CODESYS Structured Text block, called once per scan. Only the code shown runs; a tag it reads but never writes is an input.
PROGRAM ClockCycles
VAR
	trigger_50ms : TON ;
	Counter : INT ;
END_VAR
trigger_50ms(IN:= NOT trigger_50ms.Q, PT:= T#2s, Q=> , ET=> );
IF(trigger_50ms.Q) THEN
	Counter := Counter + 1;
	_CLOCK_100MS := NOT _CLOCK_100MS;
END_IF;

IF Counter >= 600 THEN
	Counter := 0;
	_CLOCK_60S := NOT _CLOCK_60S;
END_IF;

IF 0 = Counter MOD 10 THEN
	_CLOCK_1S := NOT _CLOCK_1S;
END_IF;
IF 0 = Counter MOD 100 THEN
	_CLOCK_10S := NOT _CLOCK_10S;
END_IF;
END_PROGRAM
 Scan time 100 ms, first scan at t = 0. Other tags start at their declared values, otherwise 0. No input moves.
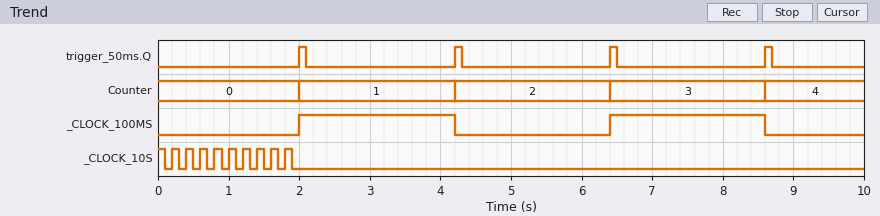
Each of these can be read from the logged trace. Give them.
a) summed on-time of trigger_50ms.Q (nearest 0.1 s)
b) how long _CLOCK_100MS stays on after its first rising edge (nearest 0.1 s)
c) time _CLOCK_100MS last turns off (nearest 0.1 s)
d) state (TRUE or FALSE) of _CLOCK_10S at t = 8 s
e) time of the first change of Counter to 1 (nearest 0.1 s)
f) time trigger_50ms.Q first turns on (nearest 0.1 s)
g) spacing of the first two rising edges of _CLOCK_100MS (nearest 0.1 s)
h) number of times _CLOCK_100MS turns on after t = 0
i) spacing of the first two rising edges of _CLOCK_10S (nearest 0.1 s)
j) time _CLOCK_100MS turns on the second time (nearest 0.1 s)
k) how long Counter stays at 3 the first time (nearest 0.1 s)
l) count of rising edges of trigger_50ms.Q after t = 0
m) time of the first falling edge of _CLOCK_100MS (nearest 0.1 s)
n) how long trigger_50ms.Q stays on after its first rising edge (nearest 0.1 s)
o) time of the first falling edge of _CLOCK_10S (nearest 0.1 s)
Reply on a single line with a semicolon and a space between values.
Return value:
0.4 s; 2.2 s; 8.6 s; FALSE; 2.0 s; 2.0 s; 4.4 s; 2; 0.2 s; 6.4 s; 2.2 s; 4; 4.2 s; 0.1 s; 0.1 s
